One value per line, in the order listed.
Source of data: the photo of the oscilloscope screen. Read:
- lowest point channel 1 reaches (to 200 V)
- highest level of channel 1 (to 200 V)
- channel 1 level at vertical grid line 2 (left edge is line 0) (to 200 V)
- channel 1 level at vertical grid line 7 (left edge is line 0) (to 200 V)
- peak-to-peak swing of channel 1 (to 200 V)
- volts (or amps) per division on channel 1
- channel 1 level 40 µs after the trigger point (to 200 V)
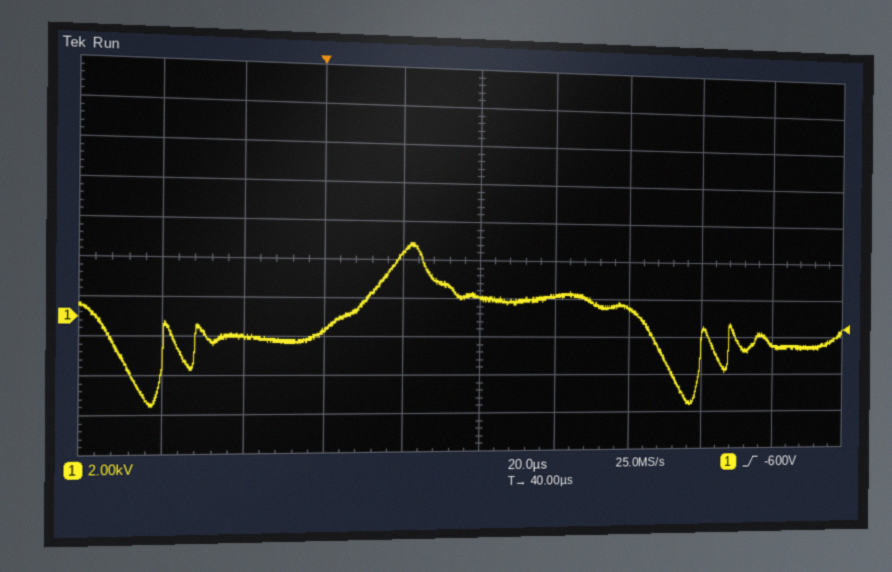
-4.6 kV
3.8 kV
-1.0 kV
600 V
8.4 kV
2 kV
1.0 kV
